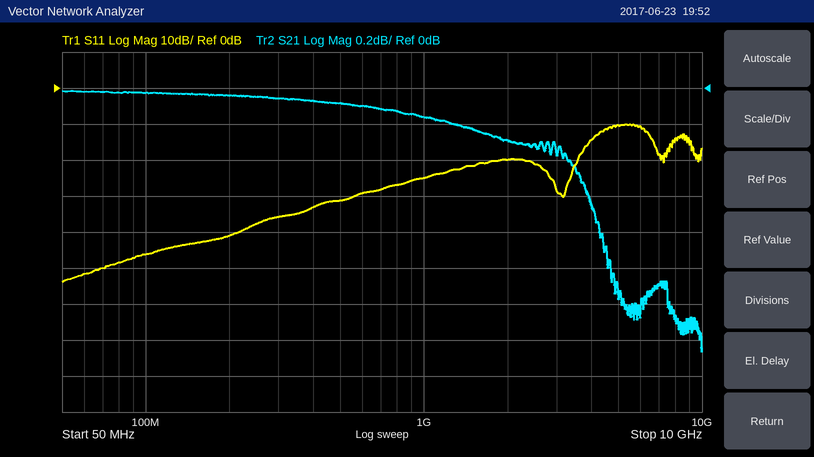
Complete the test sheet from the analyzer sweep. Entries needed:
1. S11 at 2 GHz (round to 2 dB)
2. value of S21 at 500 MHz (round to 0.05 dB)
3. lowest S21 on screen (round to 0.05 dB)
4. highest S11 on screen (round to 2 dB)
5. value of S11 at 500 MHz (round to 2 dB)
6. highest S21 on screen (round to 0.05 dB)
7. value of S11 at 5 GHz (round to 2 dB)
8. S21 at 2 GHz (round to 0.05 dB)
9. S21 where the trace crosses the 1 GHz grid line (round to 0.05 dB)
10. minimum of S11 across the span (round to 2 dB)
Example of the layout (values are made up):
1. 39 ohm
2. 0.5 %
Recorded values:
1. -20 dB
2. -0.10 dB
3. -1.45 dB
4. -10 dB
5. -32 dB
6. 0.00 dB
7. -10 dB
8. -0.30 dB
9. -0.15 dB
10. -54 dB
